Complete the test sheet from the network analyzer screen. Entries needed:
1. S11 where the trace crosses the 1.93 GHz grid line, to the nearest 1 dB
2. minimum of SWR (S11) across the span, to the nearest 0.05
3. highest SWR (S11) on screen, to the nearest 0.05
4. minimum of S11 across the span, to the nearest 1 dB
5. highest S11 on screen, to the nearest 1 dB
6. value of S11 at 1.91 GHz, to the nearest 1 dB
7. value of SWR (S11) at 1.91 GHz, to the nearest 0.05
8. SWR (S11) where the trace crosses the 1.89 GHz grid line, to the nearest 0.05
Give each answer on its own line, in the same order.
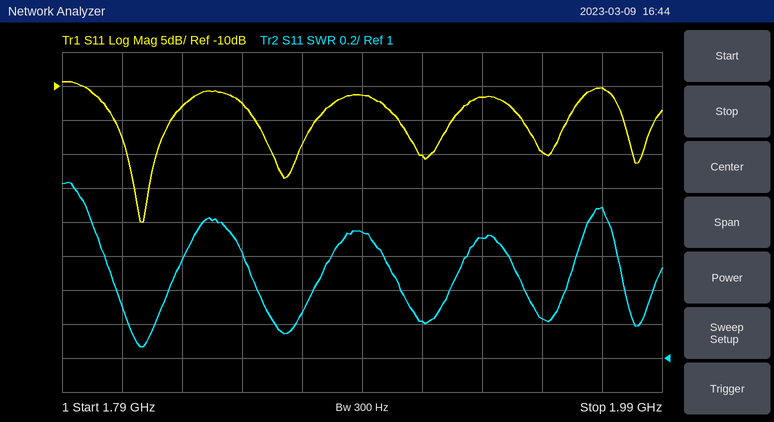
-12 dB
1.05
2.05
-30 dB
-9 dB
-20 dB
1.20
1.75
